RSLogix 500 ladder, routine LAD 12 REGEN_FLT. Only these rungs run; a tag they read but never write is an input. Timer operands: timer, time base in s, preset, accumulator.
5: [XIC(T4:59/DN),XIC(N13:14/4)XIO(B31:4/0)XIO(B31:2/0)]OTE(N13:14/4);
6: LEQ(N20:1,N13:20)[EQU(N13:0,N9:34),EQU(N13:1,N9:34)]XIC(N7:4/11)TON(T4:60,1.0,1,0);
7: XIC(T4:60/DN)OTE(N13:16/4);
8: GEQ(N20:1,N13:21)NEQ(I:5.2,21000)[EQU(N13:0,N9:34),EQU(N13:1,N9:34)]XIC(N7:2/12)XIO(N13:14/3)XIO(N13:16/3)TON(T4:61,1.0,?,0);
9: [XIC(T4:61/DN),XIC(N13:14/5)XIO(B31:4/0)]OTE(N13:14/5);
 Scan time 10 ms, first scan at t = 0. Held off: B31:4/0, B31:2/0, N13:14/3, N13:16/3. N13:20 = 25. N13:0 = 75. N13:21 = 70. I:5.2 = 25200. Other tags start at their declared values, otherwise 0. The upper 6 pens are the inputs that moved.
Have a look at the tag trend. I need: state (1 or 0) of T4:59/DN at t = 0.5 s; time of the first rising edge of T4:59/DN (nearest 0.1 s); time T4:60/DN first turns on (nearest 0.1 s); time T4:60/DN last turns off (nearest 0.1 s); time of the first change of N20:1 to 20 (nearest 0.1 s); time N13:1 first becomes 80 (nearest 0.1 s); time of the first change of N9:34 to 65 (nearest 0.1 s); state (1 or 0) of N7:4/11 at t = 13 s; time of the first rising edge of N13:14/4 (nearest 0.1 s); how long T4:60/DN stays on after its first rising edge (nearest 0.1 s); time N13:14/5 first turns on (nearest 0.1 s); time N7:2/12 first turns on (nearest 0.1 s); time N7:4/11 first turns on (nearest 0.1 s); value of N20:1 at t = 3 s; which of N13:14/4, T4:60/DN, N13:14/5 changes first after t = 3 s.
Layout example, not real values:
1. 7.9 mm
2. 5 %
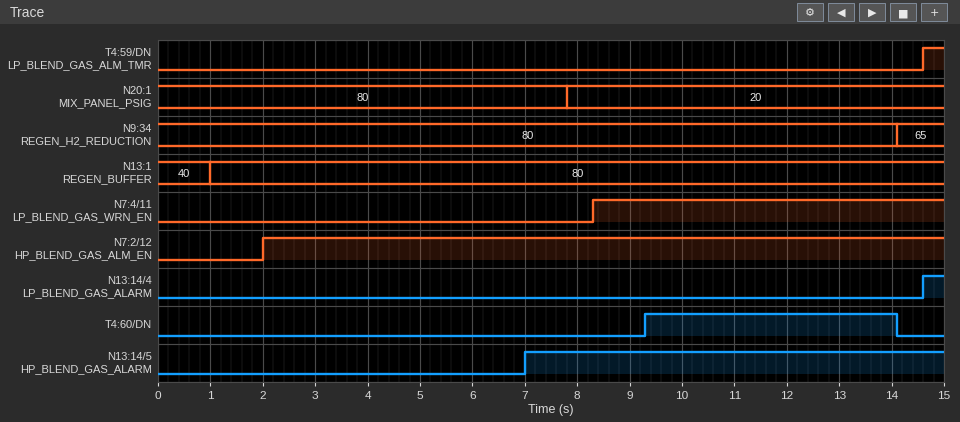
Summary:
1. 0
2. 14.6 s
3. 9.3 s
4. 14.1 s
5. 7.8 s
6. 1.0 s
7. 14.1 s
8. 1
9. 14.6 s
10. 4.8 s
11. 7.0 s
12. 2.0 s
13. 8.3 s
14. 80
15. N13:14/5
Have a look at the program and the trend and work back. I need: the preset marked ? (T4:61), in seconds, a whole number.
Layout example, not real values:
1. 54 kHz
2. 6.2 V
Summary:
1. 5 s
